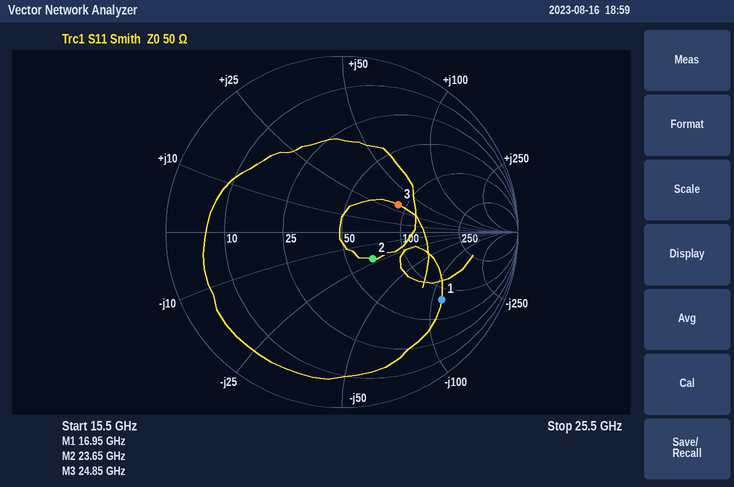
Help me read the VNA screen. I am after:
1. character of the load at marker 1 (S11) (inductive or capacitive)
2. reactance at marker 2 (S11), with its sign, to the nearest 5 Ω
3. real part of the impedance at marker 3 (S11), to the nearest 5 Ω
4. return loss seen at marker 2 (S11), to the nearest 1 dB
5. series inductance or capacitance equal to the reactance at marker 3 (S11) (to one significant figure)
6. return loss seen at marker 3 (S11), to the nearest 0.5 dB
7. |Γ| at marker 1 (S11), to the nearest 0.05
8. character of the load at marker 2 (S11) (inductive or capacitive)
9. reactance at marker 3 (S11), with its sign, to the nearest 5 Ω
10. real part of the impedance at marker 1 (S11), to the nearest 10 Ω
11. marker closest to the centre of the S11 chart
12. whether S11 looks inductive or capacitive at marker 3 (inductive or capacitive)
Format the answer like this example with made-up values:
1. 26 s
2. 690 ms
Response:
1. capacitive
2. -20 Ω
3. 90 Ω
4. 13 dB
5. 200 pH
6. 9.0 dB
7. 0.70
8. capacitive
9. +30 Ω
10. 80 Ω
11. marker 2
12. inductive
